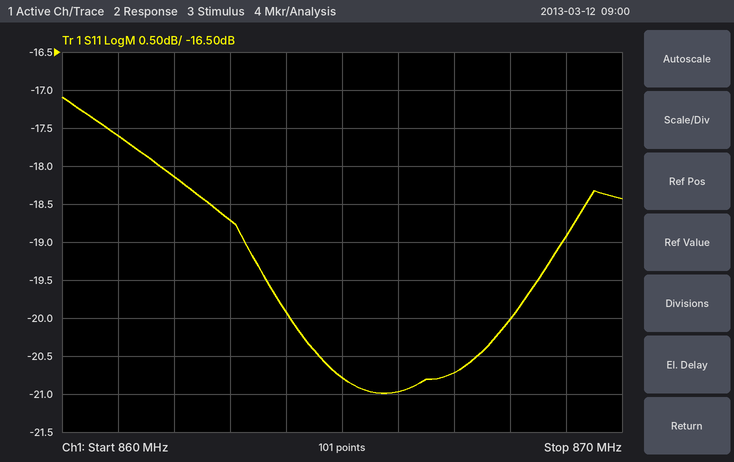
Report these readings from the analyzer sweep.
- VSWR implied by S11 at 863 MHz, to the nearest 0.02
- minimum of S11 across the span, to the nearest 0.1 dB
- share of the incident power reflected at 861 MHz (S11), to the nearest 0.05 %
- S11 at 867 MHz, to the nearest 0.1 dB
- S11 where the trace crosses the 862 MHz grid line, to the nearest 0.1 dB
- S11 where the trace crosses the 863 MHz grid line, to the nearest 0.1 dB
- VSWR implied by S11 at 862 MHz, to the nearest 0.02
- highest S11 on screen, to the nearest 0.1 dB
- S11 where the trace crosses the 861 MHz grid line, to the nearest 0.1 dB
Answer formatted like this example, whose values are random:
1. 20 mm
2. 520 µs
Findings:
1. 1.26
2. -21.0 dB
3. 1.75 %
4. -20.7 dB
5. -18.1 dB
6. -18.7 dB
7. 1.28
8. -17.1 dB
9. -17.6 dB
